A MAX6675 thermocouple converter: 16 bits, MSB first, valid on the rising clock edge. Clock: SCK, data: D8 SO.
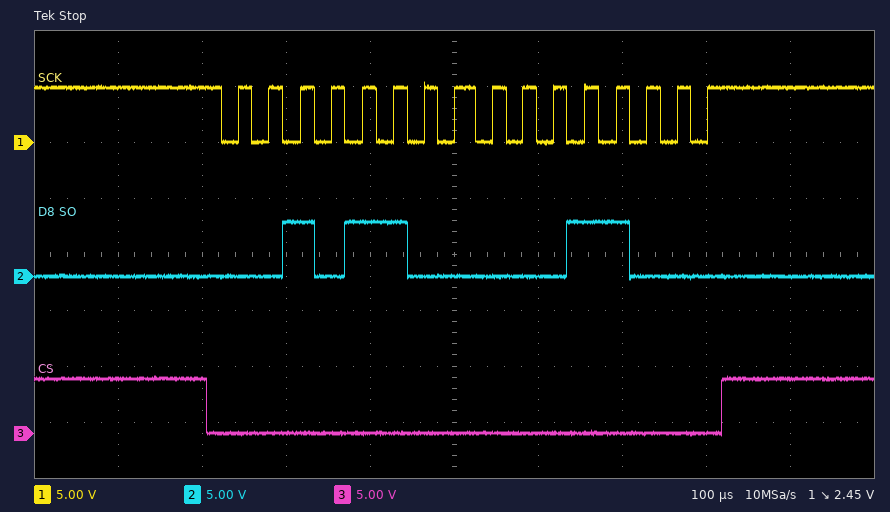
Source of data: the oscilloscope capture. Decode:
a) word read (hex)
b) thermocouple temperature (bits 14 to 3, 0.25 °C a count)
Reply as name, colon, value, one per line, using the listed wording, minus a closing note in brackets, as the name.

word read: 0x2C18
thermocouple temperature: 352.75 °C
